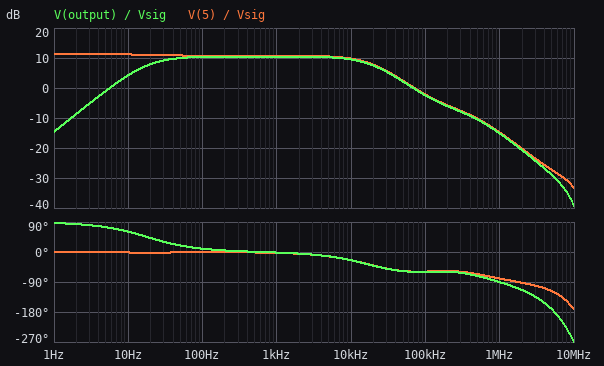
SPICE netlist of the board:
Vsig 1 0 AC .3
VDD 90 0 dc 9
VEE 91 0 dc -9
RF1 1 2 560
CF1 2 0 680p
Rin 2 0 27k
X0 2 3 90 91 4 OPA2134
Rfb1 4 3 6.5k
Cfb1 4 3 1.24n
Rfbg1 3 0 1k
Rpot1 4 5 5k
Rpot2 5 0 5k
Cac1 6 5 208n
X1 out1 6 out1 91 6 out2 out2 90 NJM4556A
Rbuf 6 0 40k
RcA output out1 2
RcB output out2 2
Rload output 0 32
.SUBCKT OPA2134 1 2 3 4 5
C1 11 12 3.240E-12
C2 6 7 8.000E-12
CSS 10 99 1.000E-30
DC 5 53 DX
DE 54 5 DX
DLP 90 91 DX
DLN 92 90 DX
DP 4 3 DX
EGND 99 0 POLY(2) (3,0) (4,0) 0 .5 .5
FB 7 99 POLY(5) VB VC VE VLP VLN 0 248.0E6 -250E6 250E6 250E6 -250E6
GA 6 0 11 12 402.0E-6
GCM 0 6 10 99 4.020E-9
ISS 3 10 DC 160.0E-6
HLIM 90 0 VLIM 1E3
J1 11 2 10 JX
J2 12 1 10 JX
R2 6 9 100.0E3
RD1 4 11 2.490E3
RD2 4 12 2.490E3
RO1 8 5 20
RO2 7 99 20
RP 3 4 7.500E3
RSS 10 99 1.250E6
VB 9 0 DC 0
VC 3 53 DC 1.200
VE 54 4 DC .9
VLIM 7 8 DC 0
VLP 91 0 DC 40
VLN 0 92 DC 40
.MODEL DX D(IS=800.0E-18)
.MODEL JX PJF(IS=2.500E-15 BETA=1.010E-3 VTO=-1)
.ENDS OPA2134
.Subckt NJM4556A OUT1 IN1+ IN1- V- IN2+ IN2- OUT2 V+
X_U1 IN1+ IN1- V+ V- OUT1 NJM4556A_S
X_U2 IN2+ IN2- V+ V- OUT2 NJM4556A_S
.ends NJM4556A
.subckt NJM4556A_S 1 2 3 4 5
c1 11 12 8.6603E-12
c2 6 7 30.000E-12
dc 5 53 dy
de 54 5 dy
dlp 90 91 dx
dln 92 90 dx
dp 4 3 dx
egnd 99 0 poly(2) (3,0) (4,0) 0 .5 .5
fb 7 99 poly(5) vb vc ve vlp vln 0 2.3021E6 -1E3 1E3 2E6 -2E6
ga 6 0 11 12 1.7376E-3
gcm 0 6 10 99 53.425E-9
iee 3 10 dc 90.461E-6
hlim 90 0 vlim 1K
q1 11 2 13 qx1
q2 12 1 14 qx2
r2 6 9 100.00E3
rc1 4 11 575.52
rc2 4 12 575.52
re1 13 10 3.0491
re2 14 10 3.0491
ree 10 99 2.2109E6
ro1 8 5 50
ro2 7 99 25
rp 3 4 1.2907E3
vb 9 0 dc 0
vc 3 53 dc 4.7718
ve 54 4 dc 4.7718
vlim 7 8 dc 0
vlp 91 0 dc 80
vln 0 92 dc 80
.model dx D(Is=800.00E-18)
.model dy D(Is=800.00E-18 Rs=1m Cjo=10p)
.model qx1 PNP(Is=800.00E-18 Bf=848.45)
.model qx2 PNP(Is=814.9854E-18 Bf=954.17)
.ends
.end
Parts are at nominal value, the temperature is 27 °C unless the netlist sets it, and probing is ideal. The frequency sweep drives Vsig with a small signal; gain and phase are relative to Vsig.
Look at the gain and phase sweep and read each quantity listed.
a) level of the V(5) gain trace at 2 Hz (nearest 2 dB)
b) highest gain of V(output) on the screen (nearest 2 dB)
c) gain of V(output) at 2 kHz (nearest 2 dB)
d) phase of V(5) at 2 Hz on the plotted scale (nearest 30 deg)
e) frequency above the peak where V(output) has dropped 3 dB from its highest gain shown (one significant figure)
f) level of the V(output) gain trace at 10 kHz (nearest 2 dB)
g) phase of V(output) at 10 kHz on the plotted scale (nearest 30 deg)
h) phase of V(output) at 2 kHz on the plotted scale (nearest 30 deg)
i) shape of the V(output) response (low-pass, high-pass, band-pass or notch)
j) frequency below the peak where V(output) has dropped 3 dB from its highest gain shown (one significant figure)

12 dB
10 dB
10 dB
0 deg
20 kHz
10 dB
-30 deg
0 deg
band-pass
20 Hz
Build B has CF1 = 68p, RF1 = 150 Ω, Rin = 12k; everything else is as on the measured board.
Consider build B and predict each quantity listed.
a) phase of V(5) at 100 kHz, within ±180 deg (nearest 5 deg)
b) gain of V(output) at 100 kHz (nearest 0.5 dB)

-45 deg
-2.0 dB
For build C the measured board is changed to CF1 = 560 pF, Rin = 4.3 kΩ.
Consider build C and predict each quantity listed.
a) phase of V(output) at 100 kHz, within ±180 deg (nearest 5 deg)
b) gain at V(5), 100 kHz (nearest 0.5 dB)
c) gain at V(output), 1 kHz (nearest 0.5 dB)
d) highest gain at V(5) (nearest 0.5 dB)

-55 deg
-3.0 dB
9.5 dB
10.5 dB
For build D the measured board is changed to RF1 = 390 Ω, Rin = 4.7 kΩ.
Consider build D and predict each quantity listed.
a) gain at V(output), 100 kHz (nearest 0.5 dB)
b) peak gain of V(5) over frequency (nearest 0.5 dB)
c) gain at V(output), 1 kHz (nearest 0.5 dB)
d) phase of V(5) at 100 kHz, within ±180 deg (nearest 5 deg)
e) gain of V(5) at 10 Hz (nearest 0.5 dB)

-3.0 dB
11.0 dB
10.0 dB
-55 deg
10.5 dB
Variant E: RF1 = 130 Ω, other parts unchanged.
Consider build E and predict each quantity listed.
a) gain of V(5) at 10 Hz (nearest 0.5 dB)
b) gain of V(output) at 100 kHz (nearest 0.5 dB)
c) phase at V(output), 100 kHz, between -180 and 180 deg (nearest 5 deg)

11.5 dB
-2.0 dB
-50 deg
